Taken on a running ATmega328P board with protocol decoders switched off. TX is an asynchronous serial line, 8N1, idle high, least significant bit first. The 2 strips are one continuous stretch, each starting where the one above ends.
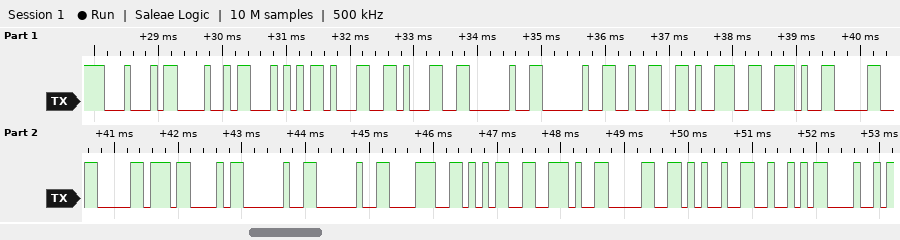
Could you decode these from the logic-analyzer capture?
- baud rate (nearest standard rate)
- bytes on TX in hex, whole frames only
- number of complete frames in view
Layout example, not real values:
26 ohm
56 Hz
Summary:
9600 baud
44 48 54 31 31 20 20 32 39 2E 30 B0 43 20 20 38 35 2E 30 25 52 48
22
